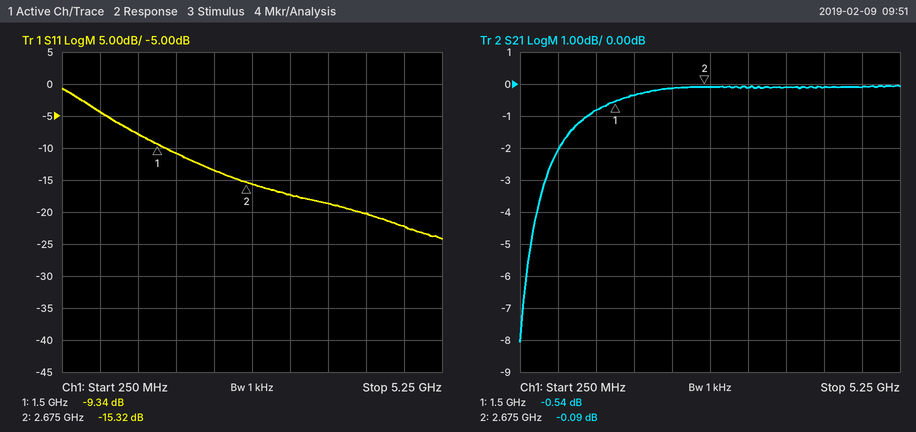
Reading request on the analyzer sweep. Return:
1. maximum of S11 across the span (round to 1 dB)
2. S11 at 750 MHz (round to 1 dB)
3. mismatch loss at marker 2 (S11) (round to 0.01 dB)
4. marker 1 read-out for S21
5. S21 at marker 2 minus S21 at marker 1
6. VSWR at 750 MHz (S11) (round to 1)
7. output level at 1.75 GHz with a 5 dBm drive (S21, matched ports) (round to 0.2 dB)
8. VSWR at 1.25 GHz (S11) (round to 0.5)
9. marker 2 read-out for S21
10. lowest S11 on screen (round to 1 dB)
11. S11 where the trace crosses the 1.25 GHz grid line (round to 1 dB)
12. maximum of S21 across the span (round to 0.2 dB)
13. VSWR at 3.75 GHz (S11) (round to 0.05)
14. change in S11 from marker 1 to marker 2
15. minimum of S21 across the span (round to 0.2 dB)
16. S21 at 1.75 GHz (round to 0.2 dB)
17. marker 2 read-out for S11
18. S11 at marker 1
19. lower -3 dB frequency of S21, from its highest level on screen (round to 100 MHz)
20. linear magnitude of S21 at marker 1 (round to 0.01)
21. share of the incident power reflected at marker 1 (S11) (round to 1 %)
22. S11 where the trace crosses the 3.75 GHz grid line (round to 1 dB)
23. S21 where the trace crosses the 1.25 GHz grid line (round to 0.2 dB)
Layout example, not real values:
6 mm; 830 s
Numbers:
-1 dB; -4 dB; 0.13 dB; -0.54 dB; 0.45 dB; 4; 4.6 dBm; 2.5; -0.09 dB; -24 dB; -8 dB; 0.0 dB; 1.25; -5.98 dB; -8.0 dB; -0.4 dB; -15.32 dB; -9.34 dB; 600 MHz; 0.94; 12 %; -19 dB; -0.8 dB
